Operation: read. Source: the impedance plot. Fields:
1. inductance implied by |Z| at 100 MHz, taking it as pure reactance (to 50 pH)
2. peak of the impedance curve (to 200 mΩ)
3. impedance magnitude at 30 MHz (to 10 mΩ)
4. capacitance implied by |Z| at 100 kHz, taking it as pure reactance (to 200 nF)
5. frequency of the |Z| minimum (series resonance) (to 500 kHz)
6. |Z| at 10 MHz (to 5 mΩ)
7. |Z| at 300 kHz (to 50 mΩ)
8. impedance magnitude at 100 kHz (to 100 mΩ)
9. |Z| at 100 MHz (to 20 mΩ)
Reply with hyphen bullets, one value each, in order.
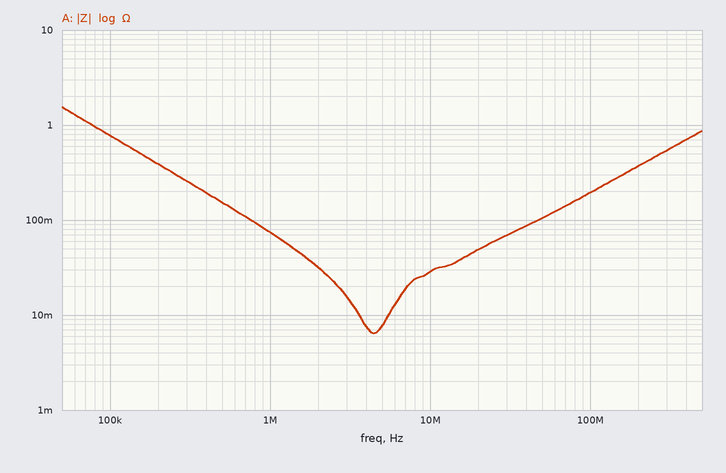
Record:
- 300 pH
- 1.6 Ω
- 70 mΩ
- 2.0 µF
- 4.5 MHz
- 30 mΩ
- 250 mΩ
- 800 mΩ
- 200 mΩ
